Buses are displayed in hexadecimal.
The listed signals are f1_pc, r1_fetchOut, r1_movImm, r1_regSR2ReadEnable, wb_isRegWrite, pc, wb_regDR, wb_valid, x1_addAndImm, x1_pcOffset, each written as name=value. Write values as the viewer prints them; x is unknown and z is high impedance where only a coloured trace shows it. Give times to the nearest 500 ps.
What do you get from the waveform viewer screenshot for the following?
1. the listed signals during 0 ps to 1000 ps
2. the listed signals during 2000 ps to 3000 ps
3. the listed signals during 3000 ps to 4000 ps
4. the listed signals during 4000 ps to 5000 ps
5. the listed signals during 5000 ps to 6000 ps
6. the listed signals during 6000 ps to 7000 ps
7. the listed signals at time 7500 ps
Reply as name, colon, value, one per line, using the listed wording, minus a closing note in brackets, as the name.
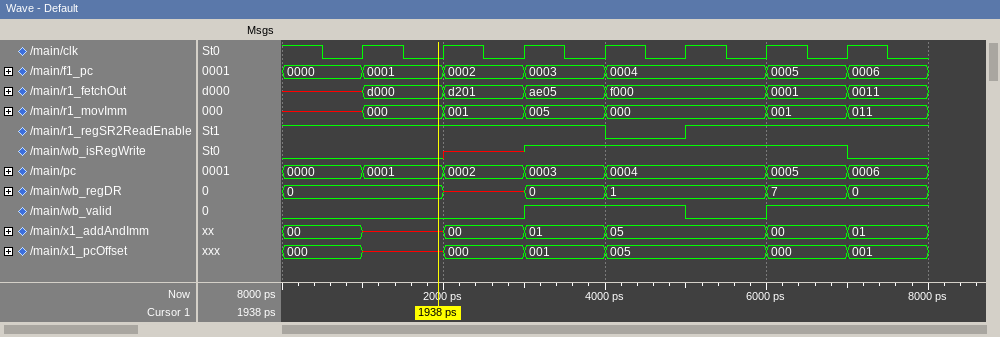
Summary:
the listed signals during 0 ps to 1000 ps: f1_pc=0000, r1_fetchOut=x, r1_movImm=x, r1_regSR2ReadEnable=1, wb_isRegWrite=0, pc=0000, wb_regDR=0, wb_valid=0, x1_addAndImm=00, x1_pcOffset=000
the listed signals during 2000 ps to 3000 ps: f1_pc=0002, r1_fetchOut=d201, r1_movImm=001, r1_regSR2ReadEnable=1, wb_isRegWrite=x, pc=0002, wb_regDR=x, wb_valid=0, x1_addAndImm=00, x1_pcOffset=000
the listed signals during 3000 ps to 4000 ps: f1_pc=0003, r1_fetchOut=ae05, r1_movImm=005, r1_regSR2ReadEnable=1, wb_isRegWrite=1, pc=0003, wb_regDR=0, wb_valid=1, x1_addAndImm=01, x1_pcOffset=001
the listed signals during 4000 ps to 5000 ps: f1_pc=0004, r1_fetchOut=f000, r1_movImm=000, r1_regSR2ReadEnable=0, wb_isRegWrite=1, pc=0004, wb_regDR=1, wb_valid=1, x1_addAndImm=05, x1_pcOffset=005
the listed signals during 5000 ps to 6000 ps: f1_pc=0004, r1_fetchOut=f000, r1_movImm=000, r1_regSR2ReadEnable=1, wb_isRegWrite=1, pc=0004, wb_regDR=1, wb_valid=0, x1_addAndImm=05, x1_pcOffset=005
the listed signals during 6000 ps to 7000 ps: f1_pc=0005, r1_fetchOut=0001, r1_movImm=001, r1_regSR2ReadEnable=1, wb_isRegWrite=1, pc=0005, wb_regDR=7, wb_valid=1, x1_addAndImm=00, x1_pcOffset=000
the listed signals at time 7500 ps: f1_pc=0006, r1_fetchOut=0011, r1_movImm=011, r1_regSR2ReadEnable=1, wb_isRegWrite=0, pc=0006, wb_regDR=0, wb_valid=1, x1_addAndImm=01, x1_pcOffset=001
